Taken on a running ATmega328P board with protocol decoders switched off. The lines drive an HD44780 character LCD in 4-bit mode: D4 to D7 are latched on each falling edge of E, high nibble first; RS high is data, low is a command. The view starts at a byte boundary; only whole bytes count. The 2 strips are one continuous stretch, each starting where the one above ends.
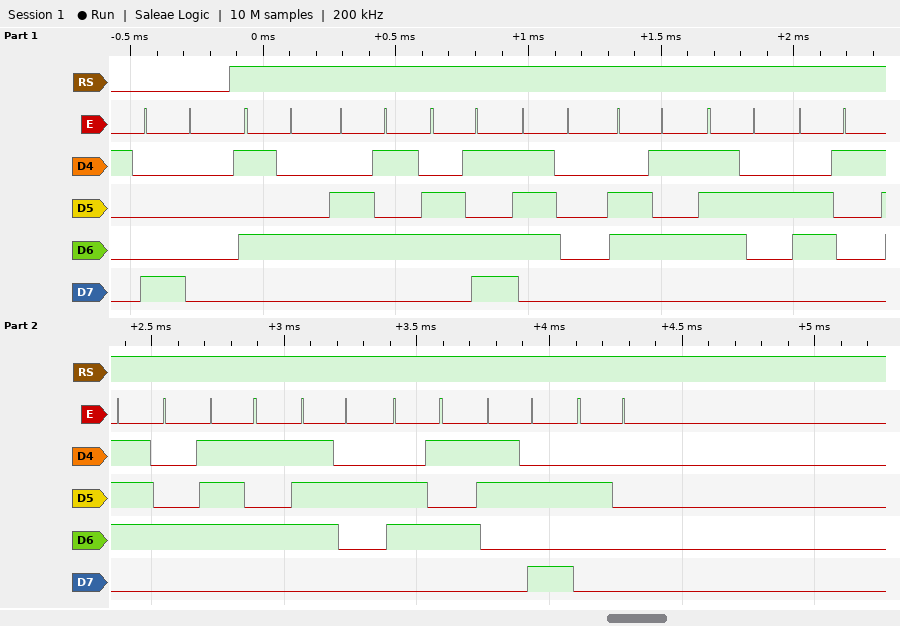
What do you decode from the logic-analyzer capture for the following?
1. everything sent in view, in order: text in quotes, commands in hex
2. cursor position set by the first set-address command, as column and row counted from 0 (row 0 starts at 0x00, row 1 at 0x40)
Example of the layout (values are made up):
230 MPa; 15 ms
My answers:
0x80 "Temperature: "; column 0, row 0
